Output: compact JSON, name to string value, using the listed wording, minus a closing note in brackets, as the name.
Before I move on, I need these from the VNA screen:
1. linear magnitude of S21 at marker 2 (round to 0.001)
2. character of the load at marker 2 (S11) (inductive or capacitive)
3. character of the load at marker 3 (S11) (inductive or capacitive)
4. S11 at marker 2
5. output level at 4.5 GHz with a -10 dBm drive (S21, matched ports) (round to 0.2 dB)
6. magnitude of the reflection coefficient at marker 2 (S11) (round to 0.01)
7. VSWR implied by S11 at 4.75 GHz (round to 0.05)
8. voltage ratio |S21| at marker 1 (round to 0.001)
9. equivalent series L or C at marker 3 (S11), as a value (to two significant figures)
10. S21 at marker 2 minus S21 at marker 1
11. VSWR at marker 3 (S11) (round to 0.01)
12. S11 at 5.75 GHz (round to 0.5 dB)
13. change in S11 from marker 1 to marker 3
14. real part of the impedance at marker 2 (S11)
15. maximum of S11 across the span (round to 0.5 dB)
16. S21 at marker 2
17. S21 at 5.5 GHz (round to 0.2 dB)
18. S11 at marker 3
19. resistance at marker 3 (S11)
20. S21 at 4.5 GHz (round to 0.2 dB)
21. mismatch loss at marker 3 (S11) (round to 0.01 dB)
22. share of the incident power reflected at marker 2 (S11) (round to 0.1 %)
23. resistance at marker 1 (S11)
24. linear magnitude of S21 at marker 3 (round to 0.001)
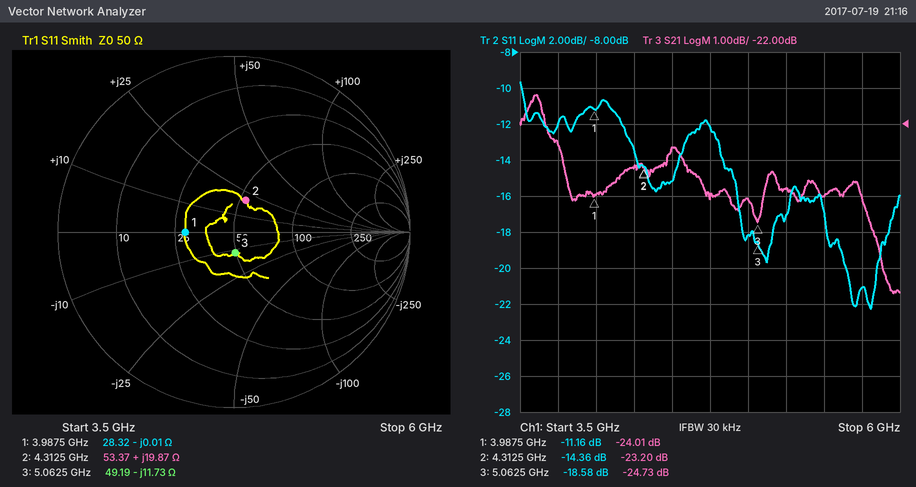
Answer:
{"linear magnitude of S21 at marker 2": "0.069", "character of the load at marker 2 (S11)": "inductive", "character of the load at marker 3 (S11)": "capacitive", "S11 at marker 2": "-14.36 dB", "output level at 4.5 GHz with a -10 dBm drive (S21, matched ports)": "-32.6 dBm", "magnitude of the reflection coefficient at marker 2 (S11)": "0.19", "VSWR implied by S11 at 4.75 GHz": "1.65", "voltage ratio |S21| at marker 1": "0.063", "equivalent series L or C at marker 3 (S11), as a value": "2.7 pF", "S21 at marker 2 minus S21 at marker 1": "0.81 dB", "VSWR at marker 3 (S11)": "1.27", "S11 at 5.75 GHz": "-21.0 dB", "change in S11 from marker 1 to marker 3": "-7.42 dB", "real part of the impedance at marker 2": "53.37 Ω", "maximum of S11 across the span": "-9.5 dB", "S21 at marker 2": "-23.20 dB", "S21 at 5.5 GHz": "-24.0 dB", "S11 at marker 3": "-18.58 dB", "resistance at marker 3": "49.19 Ω", "S21 at 4.5 GHz": "-22.6 dB", "mismatch loss at marker 3 (S11)": "0.06 dB", "share of the incident power reflected at marker 2 (S11)": "3.7 %", "resistance at marker 1": "28.32 Ω", "linear magnitude of S21 at marker 3": "0.058"}
